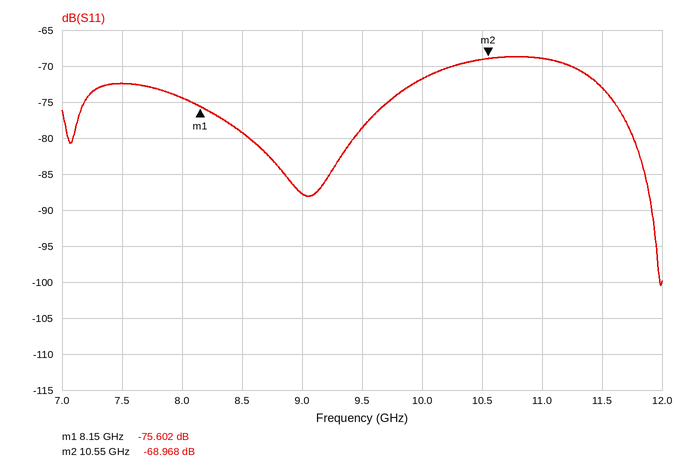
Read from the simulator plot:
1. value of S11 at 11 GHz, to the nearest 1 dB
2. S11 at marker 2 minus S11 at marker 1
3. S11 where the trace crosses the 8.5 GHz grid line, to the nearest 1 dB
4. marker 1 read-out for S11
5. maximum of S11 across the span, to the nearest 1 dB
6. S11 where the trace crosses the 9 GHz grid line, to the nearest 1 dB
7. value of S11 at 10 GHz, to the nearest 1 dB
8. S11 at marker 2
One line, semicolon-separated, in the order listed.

-69 dB; 6.634 dB; -79 dB; -75.602 dB; -69 dB; -88 dB; -72 dB; -68.968 dB
